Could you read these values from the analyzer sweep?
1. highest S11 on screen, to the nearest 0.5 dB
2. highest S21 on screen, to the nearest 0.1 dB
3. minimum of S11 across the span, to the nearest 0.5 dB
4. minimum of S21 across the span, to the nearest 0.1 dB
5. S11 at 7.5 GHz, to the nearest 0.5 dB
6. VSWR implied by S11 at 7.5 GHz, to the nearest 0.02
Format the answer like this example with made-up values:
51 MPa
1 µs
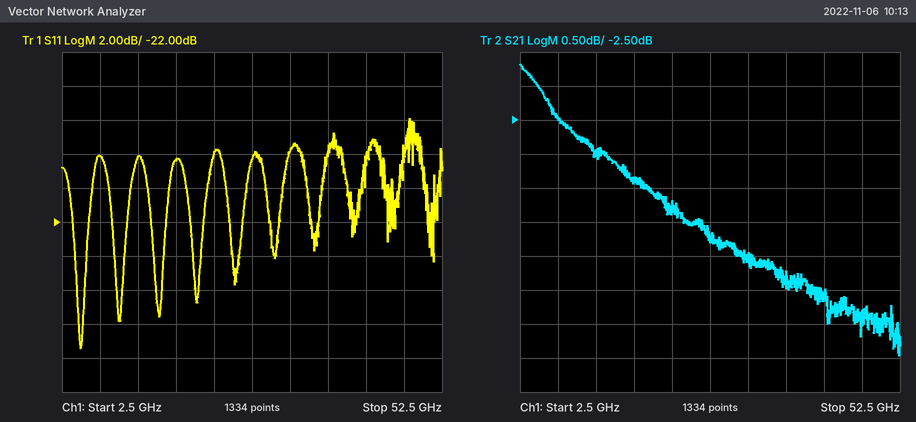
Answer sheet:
-16.0 dB
-1.7 dB
-29.5 dB
-6.0 dB
-18.0 dB
1.28
